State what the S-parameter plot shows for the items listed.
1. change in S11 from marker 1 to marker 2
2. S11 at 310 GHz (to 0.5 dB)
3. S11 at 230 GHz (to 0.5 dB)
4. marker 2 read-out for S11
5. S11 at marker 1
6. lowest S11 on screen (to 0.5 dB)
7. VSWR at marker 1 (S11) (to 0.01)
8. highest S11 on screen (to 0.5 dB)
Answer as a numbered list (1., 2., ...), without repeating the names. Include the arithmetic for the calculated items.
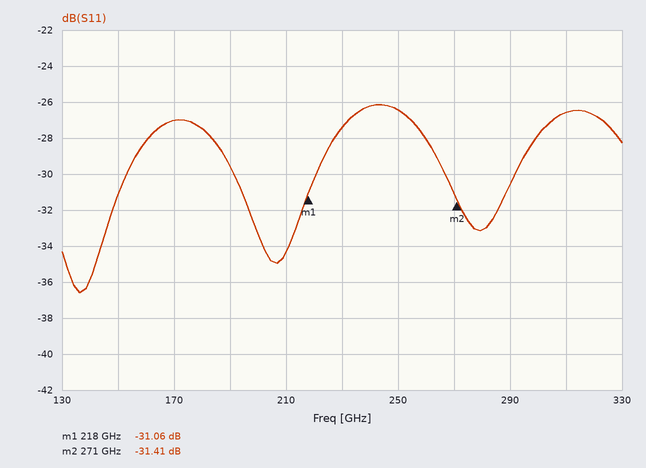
1. -31.41 − (-31.06) = -0.35 dB
2. -26.5 dB
3. -27.5 dB
4. -31.41 dB
5. -31.06 dB
6. -36.5 dB
7. (1 + 0.0280)/(1 − 0.0280) ≈ 1.06
8. -26.0 dB
